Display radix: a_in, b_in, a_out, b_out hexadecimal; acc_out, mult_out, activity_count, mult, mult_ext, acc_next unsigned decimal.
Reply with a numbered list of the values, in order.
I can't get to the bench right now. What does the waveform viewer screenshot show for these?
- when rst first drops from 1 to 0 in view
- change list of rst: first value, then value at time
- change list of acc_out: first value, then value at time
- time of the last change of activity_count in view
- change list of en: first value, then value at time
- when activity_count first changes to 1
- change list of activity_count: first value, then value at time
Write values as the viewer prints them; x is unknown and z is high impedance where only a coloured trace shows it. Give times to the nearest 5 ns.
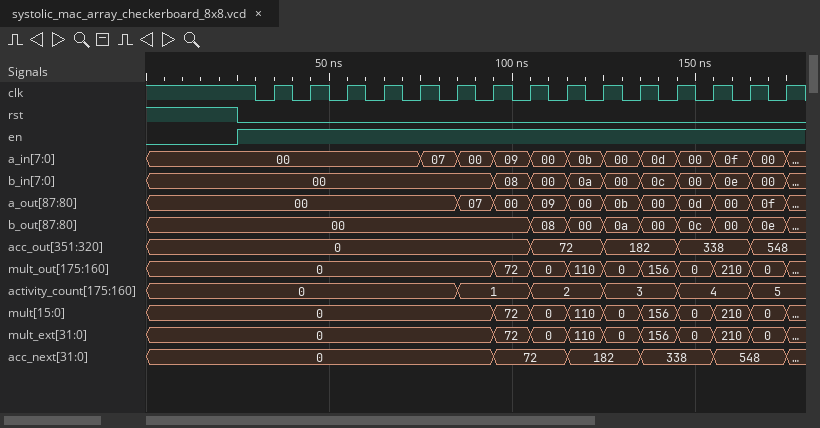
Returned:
1. 25 ns
2. 1, 0 at 25 ns
3. 0, 72 at 105 ns, 182 at 125 ns, 338 at 145 ns, 548 at 165 ns
4. 165 ns
5. 0, 1 at 25 ns
6. 85 ns
7. 0, 1 at 85 ns, 2 at 105 ns, 3 at 125 ns, 4 at 145 ns, 5 at 165 ns
